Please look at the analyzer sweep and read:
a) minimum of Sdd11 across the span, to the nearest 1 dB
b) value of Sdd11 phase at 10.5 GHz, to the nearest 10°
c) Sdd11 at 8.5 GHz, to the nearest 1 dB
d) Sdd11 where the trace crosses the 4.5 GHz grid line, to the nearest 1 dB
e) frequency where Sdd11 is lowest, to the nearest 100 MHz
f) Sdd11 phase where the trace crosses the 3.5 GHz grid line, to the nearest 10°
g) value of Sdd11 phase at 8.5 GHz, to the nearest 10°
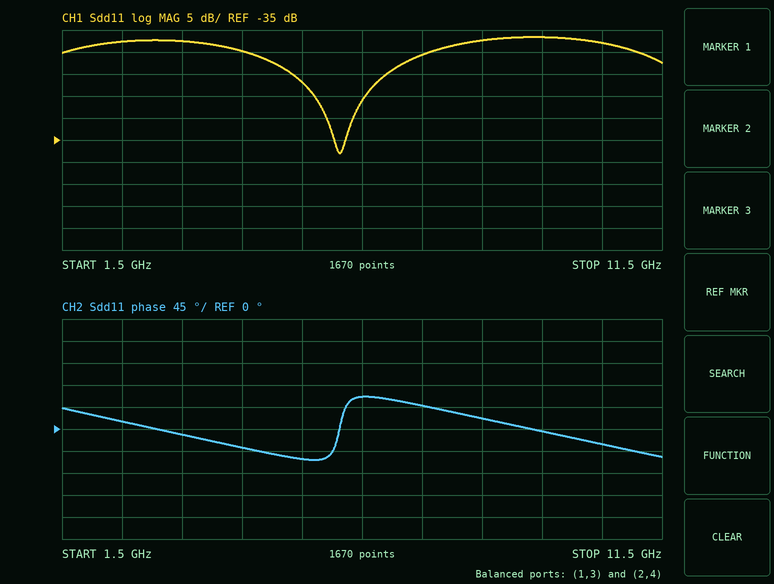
-38 dB
-30°
-12 dB
-15 dB
6.1 GHz
-10°
20°
